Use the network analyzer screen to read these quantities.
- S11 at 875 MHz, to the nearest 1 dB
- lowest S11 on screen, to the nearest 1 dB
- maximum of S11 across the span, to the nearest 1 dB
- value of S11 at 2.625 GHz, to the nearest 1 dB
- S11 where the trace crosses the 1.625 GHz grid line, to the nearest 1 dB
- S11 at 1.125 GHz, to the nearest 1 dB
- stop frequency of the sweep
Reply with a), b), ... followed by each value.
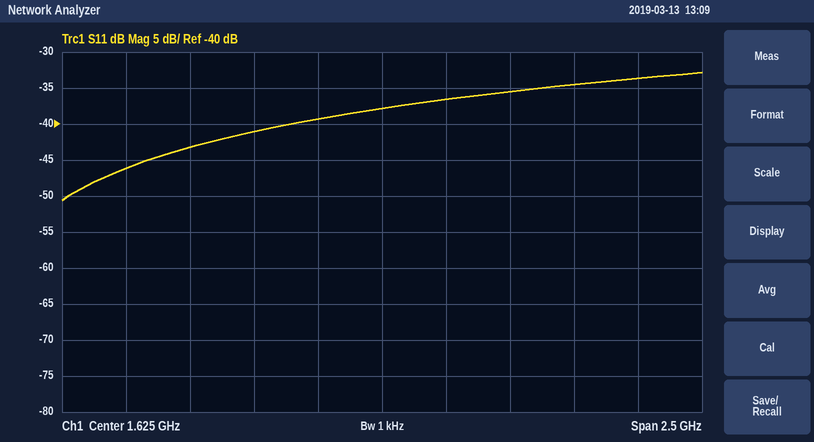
a) -43 dB
b) -51 dB
c) -33 dB
d) -34 dB
e) -38 dB
f) -41 dB
g) 2.875 GHz
